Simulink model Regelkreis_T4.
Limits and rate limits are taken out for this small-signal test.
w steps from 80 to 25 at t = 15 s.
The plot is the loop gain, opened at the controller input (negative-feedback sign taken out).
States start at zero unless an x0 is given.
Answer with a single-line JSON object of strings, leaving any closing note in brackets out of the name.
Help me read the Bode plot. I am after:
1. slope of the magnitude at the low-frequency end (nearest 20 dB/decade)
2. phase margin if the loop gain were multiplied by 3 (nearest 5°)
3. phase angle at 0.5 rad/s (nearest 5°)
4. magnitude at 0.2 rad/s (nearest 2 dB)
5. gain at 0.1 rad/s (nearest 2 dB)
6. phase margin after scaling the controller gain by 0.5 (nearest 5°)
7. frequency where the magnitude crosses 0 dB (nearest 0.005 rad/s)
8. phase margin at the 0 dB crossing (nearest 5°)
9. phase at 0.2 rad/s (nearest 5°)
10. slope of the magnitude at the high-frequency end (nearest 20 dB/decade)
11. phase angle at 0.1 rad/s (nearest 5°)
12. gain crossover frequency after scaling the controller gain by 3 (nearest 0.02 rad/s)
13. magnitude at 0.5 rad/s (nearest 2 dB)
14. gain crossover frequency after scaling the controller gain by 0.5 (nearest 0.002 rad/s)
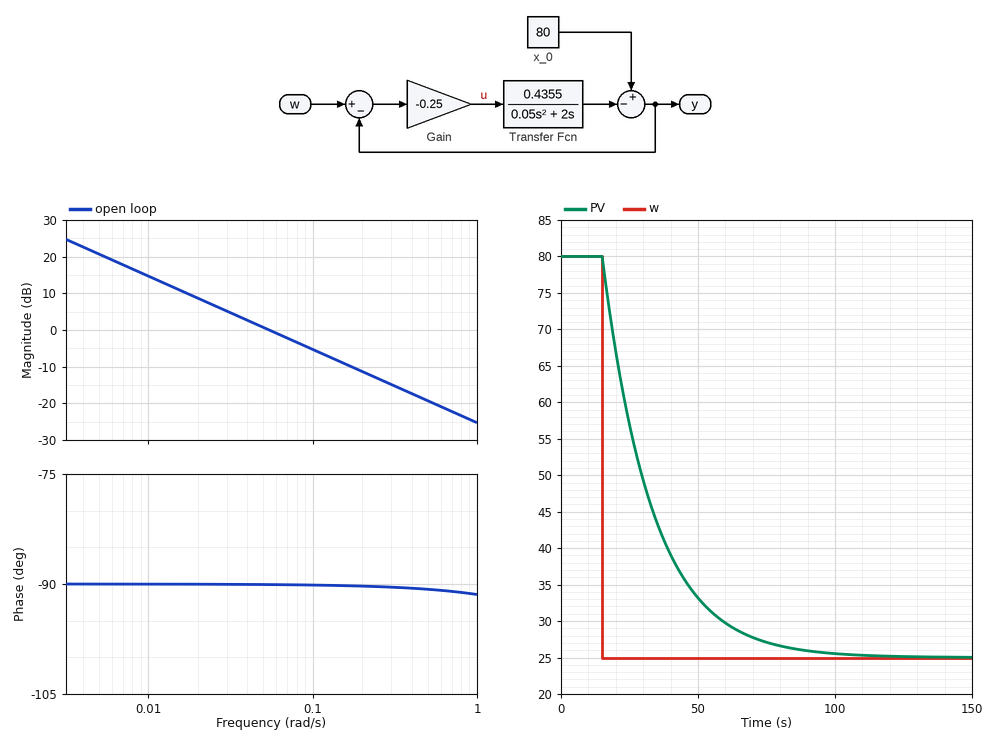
{"slope of the magnitude at the low-frequency end": "-20 dB/decade", "phase margin if the loop gain were multiplied by 3": "90°", "phase angle at 0.5 rad/s": "-90°", "magnitude at 0.2 rad/s": "-12 dB", "gain at 0.1 rad/s": "-6 dB", "phase margin after scaling the controller gain by 0.5": "90°", "frequency where the magnitude crosses 0 dB": "0.055 rad/s", "phase margin at the 0 dB crossing": "90°", "phase at 0.2 rad/s": "-90°", "slope of the magnitude at the high-frequency end": "-20 dB/decade", "phase angle at 0.1 rad/s": "-90°", "gain crossover frequency after scaling the controller gain by 3": "0.16 rad/s", "magnitude at 0.5 rad/s": "-20 dB", "gain crossover frequency after scaling the controller gain by 0.5": "0.028 rad/s"}
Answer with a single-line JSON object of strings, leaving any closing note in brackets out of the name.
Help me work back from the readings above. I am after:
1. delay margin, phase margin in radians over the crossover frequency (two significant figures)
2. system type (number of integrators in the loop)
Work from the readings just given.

{"delay margin, phase margin in radians over the crossover frequency": "29 s", "system type": "1"}
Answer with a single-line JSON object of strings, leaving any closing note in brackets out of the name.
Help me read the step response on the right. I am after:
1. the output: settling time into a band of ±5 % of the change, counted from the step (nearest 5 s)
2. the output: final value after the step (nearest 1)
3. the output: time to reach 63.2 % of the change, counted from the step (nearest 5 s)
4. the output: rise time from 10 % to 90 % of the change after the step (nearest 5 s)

{"the output: settling time into a band of ±5 % of the change, counted from the step": "55 s", "the output: final value after the step": "25", "the output: time to reach 63.2 % of the change, counted from the step": "20 s", "the output: rise time from 10 % to 90 % of the change after the step": "40 s"}
